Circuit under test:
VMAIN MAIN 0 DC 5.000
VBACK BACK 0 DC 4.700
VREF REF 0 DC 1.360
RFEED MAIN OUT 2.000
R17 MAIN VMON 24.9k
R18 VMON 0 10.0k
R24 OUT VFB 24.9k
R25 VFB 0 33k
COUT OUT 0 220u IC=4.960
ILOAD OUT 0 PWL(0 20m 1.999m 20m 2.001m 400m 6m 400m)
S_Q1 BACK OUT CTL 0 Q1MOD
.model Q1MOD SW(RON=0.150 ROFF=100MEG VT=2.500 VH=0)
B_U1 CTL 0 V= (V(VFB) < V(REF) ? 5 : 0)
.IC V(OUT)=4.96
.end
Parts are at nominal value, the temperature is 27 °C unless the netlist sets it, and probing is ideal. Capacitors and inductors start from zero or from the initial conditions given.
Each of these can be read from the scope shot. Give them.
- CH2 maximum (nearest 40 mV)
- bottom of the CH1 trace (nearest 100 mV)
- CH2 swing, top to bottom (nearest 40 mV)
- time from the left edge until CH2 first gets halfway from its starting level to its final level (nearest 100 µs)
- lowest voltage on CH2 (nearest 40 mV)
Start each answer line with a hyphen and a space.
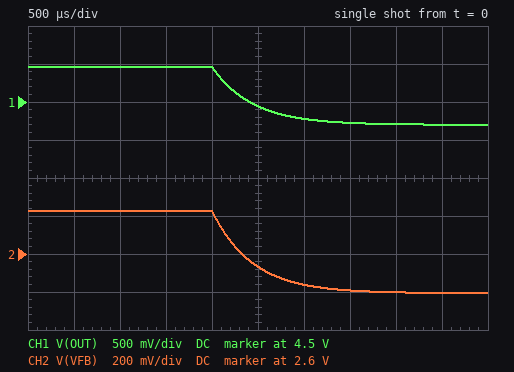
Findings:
- 2.84 V
- 4.2 V
- 440 mV
- 2.3 ms
- 2.40 V
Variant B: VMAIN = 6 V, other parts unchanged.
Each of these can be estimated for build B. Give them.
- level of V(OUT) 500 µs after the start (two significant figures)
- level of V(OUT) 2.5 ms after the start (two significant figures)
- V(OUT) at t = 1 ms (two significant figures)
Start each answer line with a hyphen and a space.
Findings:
- 5.6 V
- 5.4 V
- 5.9 V
